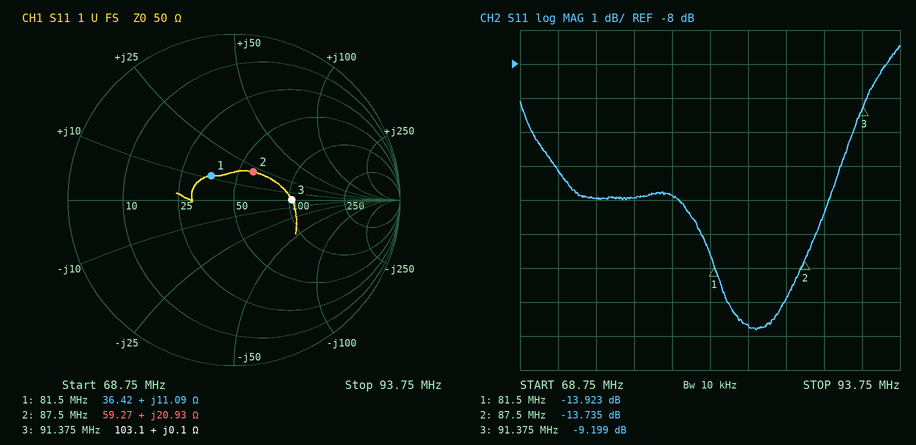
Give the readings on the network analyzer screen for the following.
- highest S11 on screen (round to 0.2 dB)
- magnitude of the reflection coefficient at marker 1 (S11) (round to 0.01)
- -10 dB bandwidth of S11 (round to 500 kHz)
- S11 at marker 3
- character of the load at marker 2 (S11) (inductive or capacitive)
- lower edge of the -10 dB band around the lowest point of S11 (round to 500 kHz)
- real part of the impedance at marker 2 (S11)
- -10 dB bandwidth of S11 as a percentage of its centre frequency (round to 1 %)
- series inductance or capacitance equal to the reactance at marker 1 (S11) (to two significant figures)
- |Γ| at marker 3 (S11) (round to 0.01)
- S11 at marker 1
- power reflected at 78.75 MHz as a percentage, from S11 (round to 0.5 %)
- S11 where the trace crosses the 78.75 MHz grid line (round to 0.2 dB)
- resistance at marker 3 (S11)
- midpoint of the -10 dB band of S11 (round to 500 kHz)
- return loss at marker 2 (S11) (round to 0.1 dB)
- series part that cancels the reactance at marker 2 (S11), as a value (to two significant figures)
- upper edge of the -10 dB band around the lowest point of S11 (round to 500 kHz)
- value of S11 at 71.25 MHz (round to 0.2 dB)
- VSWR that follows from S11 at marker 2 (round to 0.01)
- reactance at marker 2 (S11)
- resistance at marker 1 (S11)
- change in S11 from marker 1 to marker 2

-7.4 dB
0.20
21.0 MHz
-9.199 dB
inductive
69.5 MHz
59.27 Ω
26 %
22 nH
0.35
-13.923 dB
6.5 %
-11.8 dB
103.1 Ω
80.0 MHz
13.7 dB
87 pF
90.5 MHz
-11.2 dB
1.52
+20.93 Ω
36.42 Ω
0.188 dB
